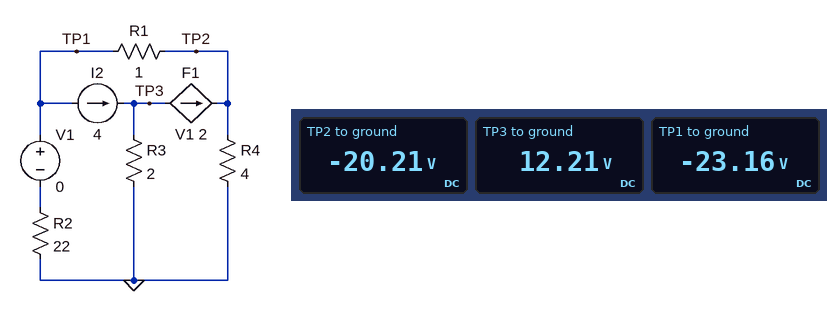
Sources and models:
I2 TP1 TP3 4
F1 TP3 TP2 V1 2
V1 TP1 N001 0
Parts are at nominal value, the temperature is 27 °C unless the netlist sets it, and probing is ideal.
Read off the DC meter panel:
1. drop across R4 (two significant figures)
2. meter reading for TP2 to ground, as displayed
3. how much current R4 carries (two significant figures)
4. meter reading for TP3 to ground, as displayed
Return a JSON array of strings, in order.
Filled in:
["20 V", "-20.21 V", "5.1 A", "12.21 V"]
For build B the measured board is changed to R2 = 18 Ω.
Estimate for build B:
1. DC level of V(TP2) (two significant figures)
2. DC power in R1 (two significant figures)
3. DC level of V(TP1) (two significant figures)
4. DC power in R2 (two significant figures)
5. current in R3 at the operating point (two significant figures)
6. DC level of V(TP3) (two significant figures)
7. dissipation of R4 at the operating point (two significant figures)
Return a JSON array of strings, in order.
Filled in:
["-21 V", "7.1 W", "-24 V", "32 W", "6.7 A", "13 V", "110 W"]
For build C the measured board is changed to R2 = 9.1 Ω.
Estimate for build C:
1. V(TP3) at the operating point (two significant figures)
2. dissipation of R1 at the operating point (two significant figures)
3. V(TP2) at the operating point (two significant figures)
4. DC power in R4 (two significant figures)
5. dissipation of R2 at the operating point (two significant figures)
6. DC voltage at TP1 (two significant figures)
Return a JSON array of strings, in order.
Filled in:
["21 V", "520 mW", "-29 V", "210 W", "98 W", "-30 V"]
